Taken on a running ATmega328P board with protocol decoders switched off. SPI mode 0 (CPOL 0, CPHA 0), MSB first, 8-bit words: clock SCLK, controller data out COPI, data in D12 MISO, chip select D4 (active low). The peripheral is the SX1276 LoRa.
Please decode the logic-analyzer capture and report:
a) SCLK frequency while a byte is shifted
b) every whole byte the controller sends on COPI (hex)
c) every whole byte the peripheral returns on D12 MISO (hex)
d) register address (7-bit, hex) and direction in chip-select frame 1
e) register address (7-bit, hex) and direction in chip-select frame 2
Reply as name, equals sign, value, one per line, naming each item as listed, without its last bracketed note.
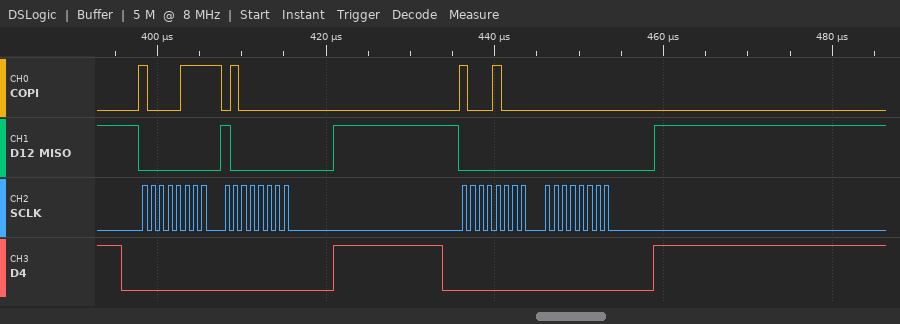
SCLK frequency while a byte is shifted = 1 MHz
every whole byte the controller sends on COPI = 0x87 0x40 0x88 0x00
every whole byte the peripheral returns on D12 MISO = 0x00 0x80 0x00 0x00
register address (7-bit, hex) and direction in chip-select frame 1 = 0x07 write
register address (7-bit, hex) and direction in chip-select frame 2 = 0x08 write
